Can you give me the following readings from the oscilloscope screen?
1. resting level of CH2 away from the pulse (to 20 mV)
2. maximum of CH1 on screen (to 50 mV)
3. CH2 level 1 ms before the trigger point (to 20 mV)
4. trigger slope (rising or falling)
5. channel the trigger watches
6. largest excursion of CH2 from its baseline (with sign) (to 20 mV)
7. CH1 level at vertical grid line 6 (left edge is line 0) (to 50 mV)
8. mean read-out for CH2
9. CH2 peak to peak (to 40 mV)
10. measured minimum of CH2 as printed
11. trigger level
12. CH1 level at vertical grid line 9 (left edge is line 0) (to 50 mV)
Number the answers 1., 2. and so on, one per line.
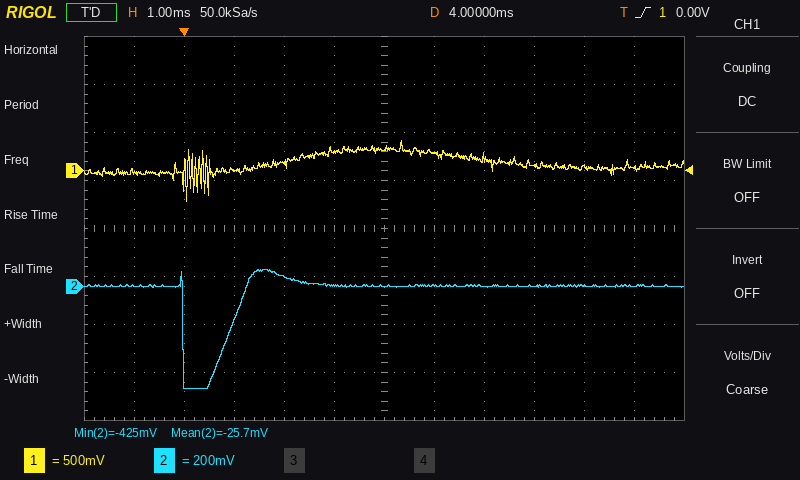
1. 0 mV
2. 300 mV
3. 0 mV
4. rising
5. CH1
6. -420 mV
7. 250 mV
8. -25.7 mV
9. 480 mV
10. -425 mV
11. 0.00 V
12. 50 mV
